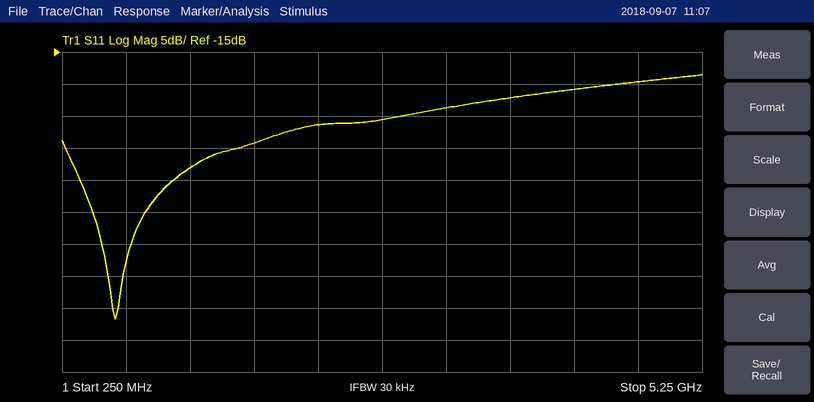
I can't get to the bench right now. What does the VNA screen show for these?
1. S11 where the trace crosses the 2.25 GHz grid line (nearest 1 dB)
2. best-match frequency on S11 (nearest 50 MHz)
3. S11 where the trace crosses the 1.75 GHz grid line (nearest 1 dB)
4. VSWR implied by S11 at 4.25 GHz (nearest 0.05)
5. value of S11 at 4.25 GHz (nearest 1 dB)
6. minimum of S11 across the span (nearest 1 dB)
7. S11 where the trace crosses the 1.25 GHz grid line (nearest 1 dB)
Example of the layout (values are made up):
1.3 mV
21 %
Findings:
-26 dB
650 MHz
-29 dB
1.20
-21 dB
-57 dB
-33 dB
